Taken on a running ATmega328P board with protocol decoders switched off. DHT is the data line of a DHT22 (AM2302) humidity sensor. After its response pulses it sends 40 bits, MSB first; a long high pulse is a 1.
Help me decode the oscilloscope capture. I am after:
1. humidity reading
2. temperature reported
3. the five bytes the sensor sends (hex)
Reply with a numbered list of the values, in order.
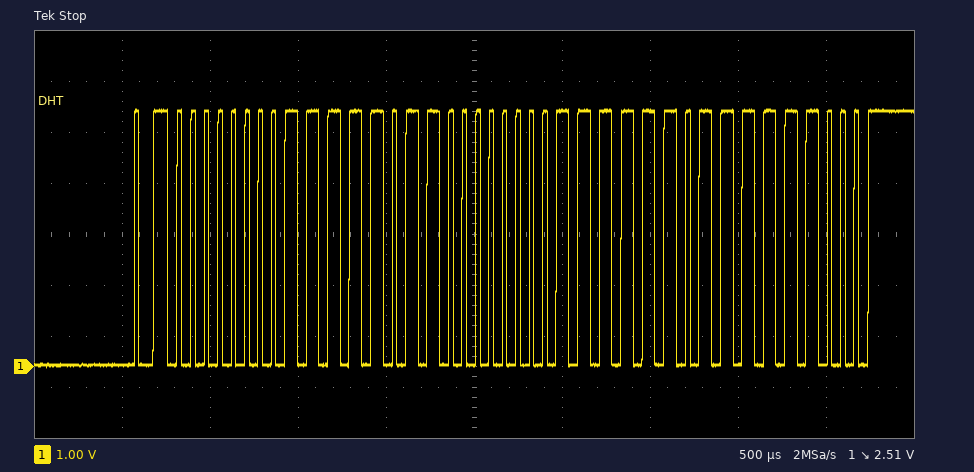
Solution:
1. 25.1 %
2. 25.3 °C
3. 00 FB 00 FD F8
